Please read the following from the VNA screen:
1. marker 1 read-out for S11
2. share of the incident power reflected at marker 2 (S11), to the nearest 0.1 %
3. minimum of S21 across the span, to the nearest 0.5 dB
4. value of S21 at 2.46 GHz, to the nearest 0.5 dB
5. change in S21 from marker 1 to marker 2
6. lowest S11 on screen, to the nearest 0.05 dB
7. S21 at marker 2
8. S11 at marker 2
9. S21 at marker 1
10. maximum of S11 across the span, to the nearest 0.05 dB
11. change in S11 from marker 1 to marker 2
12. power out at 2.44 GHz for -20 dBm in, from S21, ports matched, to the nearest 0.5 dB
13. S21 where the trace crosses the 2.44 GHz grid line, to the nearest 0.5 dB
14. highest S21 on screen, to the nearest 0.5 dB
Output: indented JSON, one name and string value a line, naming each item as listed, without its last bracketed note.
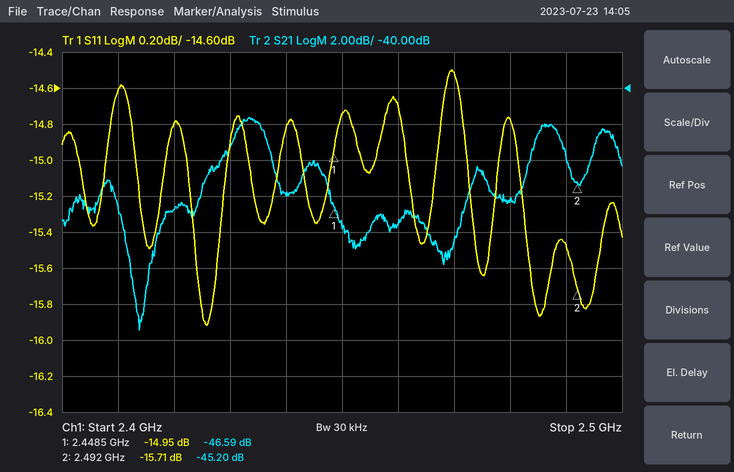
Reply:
{
  "marker 1 read-out for S11": "-14.95 dB",
  "share of the incident power reflected at marker 2 (S11), to the nearest 0.1 %": "2.7 %",
  "minimum of S21 across the span, to the nearest 0.5 dB": "-53.5 dB",
  "value of S21 at 2.46 GHz, to the nearest 0.5 dB": "-47.5 dB",
  "change in S21 from marker 1 to marker 2": "1.39 dB",
  "lowest S11 on screen, to the nearest 0.05 dB": "-15.90 dB",
  "S21 at marker 2": "-45.20 dB",
  "S11 at marker 2": "-15.71 dB",
  "S21 at marker 1": "-46.59 dB",
  "maximum of S11 across the span, to the nearest 0.05 dB": "-14.50 dB",
  "change in S11 from marker 1 to marker 2": "-0.76 dB",
  "power out at 2.44 GHz for -20 dBm in, from S21, ports matched, to the nearest 0.5 dB": "-66.0 dBm",
  "S21 where the trace crosses the 2.44 GHz grid line, to the nearest 0.5 dB": "-46.0 dB",
  "highest S21 on screen, to the nearest 0.5 dB": "-41.5 dB"
}
